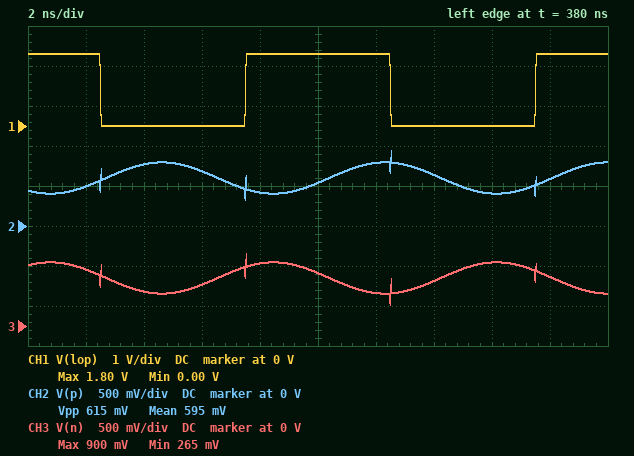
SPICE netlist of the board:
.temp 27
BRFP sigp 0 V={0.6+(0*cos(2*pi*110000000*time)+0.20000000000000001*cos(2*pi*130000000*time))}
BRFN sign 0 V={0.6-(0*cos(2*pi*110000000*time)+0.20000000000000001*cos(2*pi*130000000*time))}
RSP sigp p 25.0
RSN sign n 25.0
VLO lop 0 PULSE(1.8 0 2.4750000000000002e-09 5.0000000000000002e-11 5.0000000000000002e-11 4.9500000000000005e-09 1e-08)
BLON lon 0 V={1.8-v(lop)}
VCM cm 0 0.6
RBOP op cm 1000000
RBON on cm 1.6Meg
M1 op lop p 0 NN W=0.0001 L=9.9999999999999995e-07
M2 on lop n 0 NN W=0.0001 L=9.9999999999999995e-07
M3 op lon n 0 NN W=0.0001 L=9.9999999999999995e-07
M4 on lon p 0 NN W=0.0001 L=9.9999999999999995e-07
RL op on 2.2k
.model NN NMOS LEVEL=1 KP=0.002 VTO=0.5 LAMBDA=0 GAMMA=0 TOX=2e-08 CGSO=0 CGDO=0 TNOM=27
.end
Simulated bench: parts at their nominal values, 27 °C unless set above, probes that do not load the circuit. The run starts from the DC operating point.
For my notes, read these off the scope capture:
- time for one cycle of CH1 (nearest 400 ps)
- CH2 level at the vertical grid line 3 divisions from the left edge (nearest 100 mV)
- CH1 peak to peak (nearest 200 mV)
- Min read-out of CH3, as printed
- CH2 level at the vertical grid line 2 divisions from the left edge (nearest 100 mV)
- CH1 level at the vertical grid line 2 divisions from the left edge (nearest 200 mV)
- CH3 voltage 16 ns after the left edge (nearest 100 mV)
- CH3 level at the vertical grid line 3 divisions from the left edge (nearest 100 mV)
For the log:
10.0 ns
700 mV
1.8 V
265 mV
800 mV
0 V
800 mV
500 mV
